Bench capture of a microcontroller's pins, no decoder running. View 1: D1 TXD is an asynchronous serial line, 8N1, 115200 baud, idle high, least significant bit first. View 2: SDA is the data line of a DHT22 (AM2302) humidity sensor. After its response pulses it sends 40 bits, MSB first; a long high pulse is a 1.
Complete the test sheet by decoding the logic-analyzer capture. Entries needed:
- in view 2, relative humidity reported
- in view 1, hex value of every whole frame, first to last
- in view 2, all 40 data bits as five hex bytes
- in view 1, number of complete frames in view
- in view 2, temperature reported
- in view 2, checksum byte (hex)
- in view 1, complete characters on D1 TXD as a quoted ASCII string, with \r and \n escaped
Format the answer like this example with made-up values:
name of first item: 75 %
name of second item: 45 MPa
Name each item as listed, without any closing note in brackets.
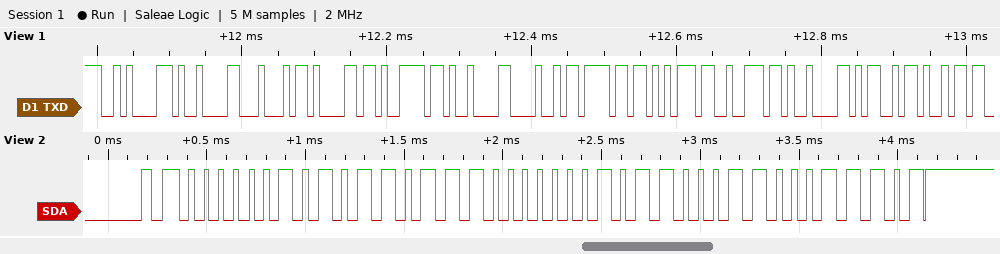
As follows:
in view 2, relative humidity reported: 69.5 %
in view 1, hex value of every whole frame, first to last: 0x0A 0x09 0x44 0x61 0x79 0x09 0x48 0x6F 0x75 0x72 0x09 0x4D 0x69
in view 2, all 40 data bits as five hex bytes: 02 B7 01 63 1D
in view 1, number of complete frames in view: 13
in view 2, temperature reported: 35.5 °C
in view 2, checksum byte: 0x1D
in view 1, complete characters on D1 TXD as a quoted ASCII string, with \r and \n escaped: "\n\tDay\tHour\tMi"
